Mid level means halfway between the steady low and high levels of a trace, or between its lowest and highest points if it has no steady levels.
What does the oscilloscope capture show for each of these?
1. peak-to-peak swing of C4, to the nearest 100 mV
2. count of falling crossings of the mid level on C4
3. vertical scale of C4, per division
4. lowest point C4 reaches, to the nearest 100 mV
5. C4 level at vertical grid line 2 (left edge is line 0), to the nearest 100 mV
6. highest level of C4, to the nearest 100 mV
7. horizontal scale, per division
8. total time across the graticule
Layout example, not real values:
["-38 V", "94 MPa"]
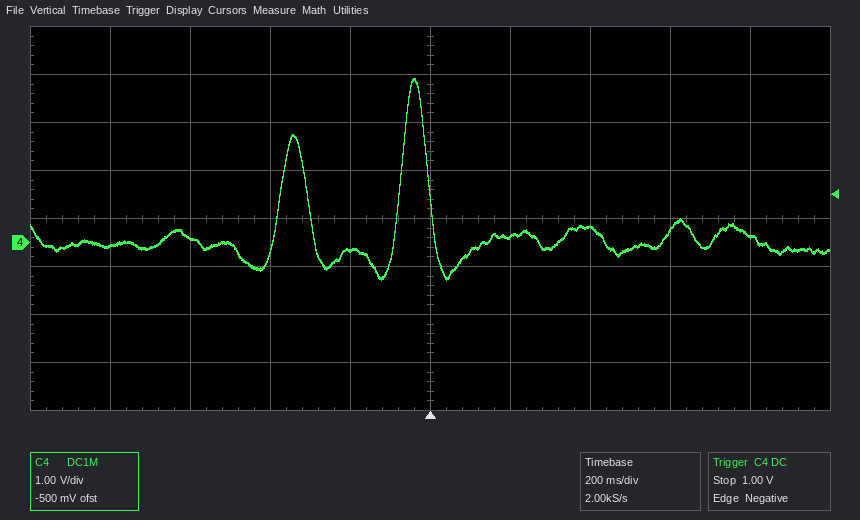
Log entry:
["4.2 V", "2", "1 V", "-800 mV", "100 mV", "3.4 V", "200 ms", "2 s"]
